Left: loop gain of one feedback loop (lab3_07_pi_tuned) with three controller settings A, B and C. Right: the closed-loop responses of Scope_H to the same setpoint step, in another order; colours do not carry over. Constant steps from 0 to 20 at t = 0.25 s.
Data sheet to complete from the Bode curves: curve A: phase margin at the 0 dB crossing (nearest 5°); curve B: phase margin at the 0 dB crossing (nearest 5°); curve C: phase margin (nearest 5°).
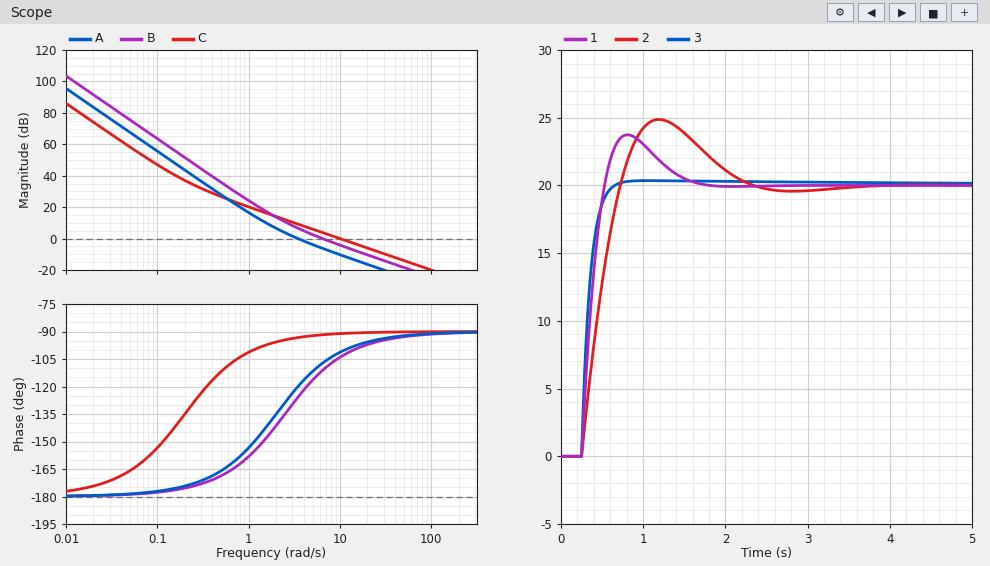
60°
70°
90°
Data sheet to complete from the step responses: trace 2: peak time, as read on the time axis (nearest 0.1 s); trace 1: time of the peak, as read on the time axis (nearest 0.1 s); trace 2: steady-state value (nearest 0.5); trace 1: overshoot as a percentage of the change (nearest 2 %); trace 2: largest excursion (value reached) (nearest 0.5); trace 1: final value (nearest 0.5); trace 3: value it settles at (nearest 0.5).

1.2 s
0.8 s
20.0
18 %
25.0
20.0
20.0
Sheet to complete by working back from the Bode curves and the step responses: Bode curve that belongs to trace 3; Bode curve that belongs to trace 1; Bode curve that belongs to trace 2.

C
B
A
